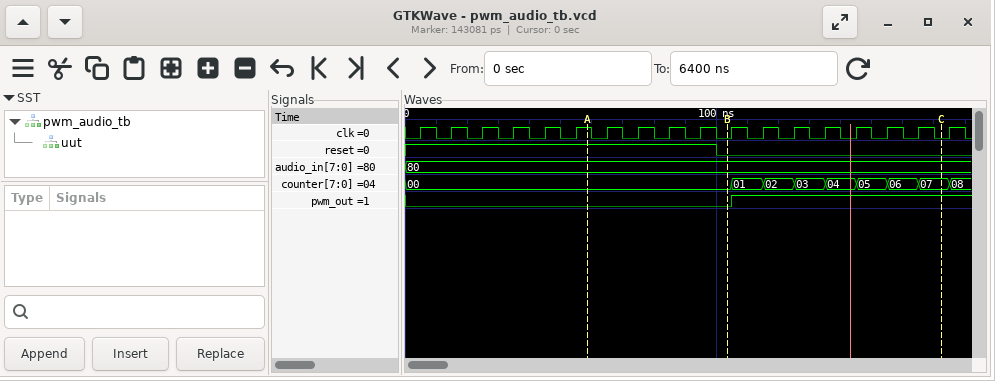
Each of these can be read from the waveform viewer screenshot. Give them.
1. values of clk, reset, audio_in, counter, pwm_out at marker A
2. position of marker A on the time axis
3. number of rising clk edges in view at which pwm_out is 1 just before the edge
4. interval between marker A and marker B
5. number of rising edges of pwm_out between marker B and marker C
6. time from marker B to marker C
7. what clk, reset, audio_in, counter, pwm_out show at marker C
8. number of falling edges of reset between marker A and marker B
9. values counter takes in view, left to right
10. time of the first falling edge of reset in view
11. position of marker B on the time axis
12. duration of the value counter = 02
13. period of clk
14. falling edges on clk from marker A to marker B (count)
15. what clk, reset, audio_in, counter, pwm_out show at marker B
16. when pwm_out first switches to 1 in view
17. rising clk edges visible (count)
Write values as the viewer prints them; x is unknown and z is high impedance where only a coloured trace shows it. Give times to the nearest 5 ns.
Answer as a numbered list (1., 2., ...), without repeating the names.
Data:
1. clk=1, reset=1, audio_in=80, counter=00, pwm_out=0
2. 60 ns
3. 7
4. 45 ns
5. 1
6. 70 ns
7. clk=0, reset=0, audio_in=80, counter=07, pwm_out=1
8. 1
9. 00, 01, 02, 03, 04, 05, 06, 07, 08
10. 100 ns
11. 105 ns
12. 10 ns
13. 10 ns
14. 5
15. clk=0, reset=0, audio_in=80, counter=00, pwm_out=0
16. 105 ns
17. 18
